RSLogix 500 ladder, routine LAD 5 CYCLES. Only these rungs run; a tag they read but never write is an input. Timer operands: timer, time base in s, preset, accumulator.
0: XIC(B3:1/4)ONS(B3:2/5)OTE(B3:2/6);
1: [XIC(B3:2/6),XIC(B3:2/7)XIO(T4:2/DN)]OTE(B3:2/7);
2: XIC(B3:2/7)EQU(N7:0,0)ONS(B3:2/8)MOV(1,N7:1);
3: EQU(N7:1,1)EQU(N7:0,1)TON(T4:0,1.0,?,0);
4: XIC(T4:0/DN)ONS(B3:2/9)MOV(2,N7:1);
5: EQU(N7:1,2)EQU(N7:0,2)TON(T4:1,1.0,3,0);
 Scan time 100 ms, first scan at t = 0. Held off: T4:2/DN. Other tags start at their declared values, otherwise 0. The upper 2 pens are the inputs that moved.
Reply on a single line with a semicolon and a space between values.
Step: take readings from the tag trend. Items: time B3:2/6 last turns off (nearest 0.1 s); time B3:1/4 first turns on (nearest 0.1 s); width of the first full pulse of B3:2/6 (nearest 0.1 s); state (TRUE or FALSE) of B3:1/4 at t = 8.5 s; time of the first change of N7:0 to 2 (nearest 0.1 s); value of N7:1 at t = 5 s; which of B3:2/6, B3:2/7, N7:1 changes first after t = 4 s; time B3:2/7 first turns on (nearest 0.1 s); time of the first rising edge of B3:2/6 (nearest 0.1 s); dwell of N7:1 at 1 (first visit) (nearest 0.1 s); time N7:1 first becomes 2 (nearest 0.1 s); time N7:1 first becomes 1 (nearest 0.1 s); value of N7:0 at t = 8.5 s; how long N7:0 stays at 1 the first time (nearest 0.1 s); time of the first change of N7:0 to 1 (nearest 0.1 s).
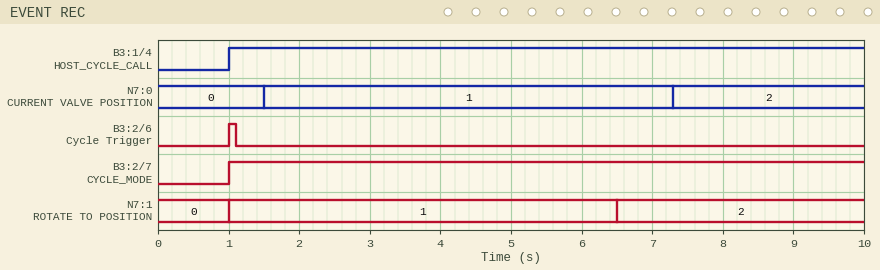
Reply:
1.1 s; 1.0 s; 0.1 s; TRUE; 7.3 s; 1; N7:1; 1.0 s; 1.0 s; 5.5 s; 6.5 s; 1.0 s; 2; 5.8 s; 1.5 s
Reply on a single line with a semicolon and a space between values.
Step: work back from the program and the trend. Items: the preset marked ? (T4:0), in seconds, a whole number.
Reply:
5 s
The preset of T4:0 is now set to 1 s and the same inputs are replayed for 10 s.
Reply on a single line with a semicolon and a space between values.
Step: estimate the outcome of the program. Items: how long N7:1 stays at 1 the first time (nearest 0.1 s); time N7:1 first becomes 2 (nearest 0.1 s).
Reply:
1.5 s; 2.5 s
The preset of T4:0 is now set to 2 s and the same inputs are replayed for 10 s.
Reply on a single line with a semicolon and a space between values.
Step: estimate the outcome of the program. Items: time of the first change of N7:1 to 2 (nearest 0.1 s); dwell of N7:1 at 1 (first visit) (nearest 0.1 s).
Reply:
3.5 s; 2.5 s
